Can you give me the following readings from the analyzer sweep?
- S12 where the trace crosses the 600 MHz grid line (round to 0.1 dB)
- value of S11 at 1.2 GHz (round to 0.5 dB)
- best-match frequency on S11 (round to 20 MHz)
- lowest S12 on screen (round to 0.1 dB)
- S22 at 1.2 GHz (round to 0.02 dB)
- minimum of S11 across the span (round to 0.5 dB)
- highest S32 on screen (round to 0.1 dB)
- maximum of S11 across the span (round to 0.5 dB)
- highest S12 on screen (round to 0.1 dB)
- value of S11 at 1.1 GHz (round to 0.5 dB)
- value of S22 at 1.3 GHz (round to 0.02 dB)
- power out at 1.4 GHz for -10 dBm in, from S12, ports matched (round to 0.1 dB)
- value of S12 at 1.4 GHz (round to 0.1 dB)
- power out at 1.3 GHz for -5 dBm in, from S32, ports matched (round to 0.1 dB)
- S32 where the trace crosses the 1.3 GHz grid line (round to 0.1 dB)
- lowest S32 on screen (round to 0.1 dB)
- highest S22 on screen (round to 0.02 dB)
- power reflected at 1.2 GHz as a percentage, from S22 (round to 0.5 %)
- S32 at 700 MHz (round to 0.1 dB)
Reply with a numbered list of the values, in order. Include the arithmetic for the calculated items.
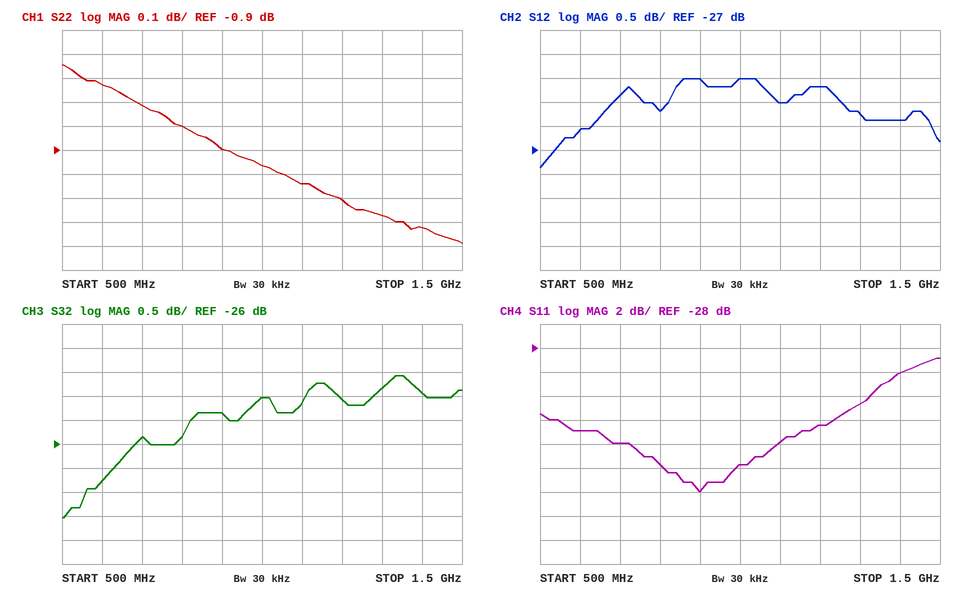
1. -26.6 dB
2. -34.5 dB
3. 900 MHz
4. -27.4 dB
5. -1.10 dB
6. -40.0 dB
7. -24.6 dB
8. -29.0 dB
9. -25.5 dB
10. -36.0 dB
11. -1.18 dB
12. -10 dBm + (-26.4 dB) = -36.4 dBm
13. -26.4 dB
14. -5 dBm + (-24.8 dB) = -29.8 dBm
15. -24.8 dB
16. -27.5 dB
17. -0.54 dB
18. 10^(-1.1/10) ≈ 77.6 %, so 77.5 % to the nearest 0.5 %
19. -25.9 dB
